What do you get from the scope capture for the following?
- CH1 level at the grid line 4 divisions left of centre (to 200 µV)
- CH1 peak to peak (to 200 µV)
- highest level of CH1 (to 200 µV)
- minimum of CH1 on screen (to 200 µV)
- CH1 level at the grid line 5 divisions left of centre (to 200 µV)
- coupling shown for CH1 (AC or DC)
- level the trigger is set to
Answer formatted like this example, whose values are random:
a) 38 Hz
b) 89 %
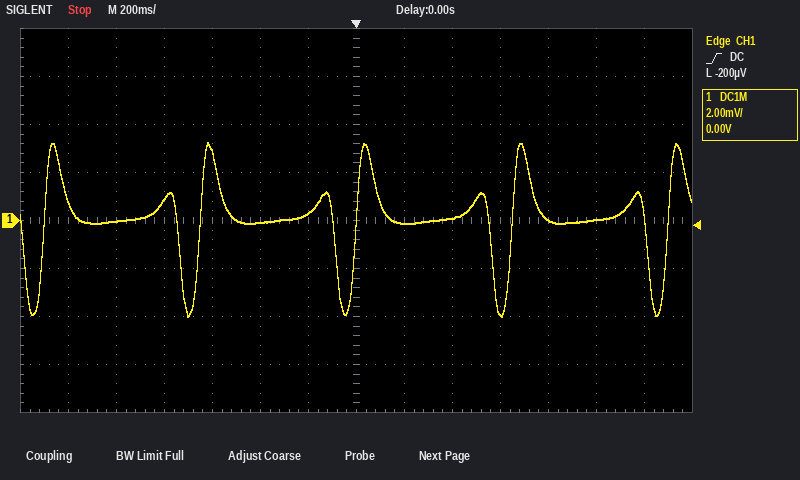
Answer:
a) 800 µV
b) 7.2 mV
c) 3.2 mV
d) -4.0 mV
e) 0.0 mV
f) DC
g) -200 µV
